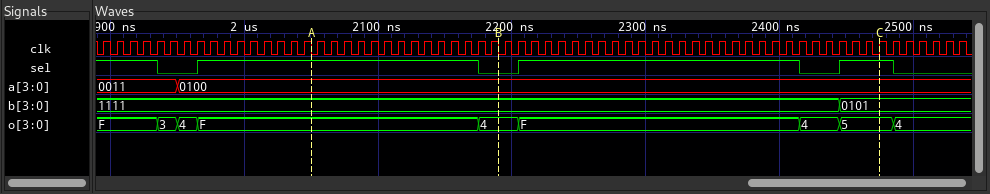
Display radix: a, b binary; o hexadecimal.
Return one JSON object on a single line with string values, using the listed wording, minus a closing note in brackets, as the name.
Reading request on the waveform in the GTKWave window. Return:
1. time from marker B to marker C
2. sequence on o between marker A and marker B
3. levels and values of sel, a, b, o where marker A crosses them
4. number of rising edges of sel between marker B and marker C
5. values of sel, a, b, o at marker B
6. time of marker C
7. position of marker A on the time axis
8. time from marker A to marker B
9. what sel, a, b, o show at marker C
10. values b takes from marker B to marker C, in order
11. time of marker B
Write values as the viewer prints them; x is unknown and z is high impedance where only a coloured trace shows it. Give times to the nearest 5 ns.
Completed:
{"time from marker B to marker C": "285 ns", "sequence on o between marker A and marker B": "F, 4", "levels and values of sel, a, b, o where marker A crosses them": "sel=1, a=0100, b=1111, o=F", "number of rising edges of sel between marker B and marker C": "2", "values of sel, a, b, o at marker B": "sel=0, a=0100, b=1111, o=4", "time of marker C": "2475 ns", "position of marker A on the time axis": "2050 ns", "time from marker A to marker B": "140 ns", "what sel, a, b, o show at marker C": "sel=1, a=0100, b=0101, o=5", "values b takes from marker B to marker C, in order": "1111, 0101", "time of marker B": "2190 ns"}
